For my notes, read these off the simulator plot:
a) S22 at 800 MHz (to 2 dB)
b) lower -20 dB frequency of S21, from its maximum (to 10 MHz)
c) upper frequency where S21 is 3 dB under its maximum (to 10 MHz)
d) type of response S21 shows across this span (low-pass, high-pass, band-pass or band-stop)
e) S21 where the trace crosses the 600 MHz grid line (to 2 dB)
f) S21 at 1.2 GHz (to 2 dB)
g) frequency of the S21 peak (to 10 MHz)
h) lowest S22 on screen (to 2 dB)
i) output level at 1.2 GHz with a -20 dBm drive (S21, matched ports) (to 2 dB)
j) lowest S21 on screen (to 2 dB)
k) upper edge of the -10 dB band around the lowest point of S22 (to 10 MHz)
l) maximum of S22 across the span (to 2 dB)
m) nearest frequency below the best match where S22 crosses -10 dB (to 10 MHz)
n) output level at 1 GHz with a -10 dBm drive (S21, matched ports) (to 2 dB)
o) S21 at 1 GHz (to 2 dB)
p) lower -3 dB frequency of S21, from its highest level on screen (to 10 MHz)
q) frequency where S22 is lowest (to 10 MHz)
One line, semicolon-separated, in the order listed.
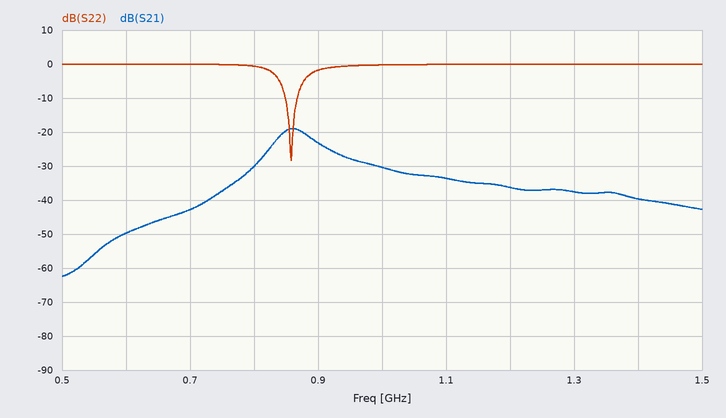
0 dB; 740 MHz; 890 MHz; band-pass; -50 dB; -36 dB; 860 MHz; -28 dB; -56 dBm; -62 dB; 870 MHz; 0 dB; 850 MHz; -40 dBm; -30 dB; 840 MHz; 860 MHz
